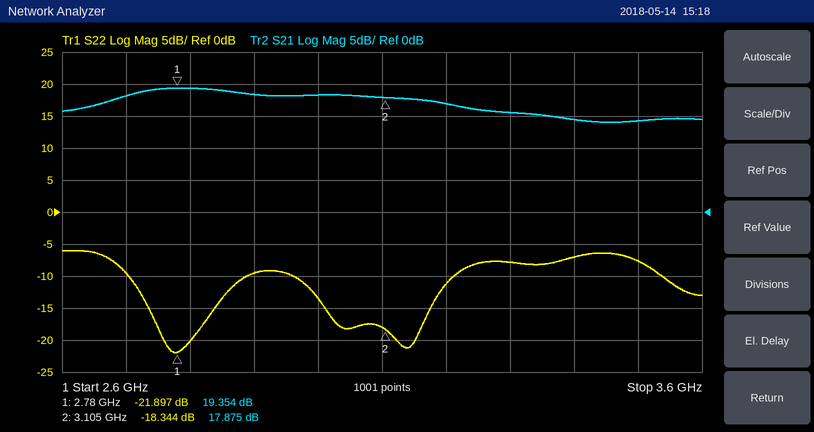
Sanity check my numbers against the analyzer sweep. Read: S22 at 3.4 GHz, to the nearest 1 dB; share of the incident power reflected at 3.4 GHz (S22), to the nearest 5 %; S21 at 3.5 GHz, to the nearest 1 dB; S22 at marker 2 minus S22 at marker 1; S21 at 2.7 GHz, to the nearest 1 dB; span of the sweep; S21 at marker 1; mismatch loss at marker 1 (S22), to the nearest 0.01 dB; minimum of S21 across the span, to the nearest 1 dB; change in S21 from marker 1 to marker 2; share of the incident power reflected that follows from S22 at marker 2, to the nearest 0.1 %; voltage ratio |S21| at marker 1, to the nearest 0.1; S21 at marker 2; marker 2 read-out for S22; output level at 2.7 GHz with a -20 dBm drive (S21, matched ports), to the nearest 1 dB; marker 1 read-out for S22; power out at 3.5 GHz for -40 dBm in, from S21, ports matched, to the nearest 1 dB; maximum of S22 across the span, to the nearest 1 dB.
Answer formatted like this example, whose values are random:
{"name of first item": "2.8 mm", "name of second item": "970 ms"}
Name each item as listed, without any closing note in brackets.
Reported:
{"S22 at 3.4 GHz, to the nearest 1 dB": "-7 dB", "share of the incident power reflected at 3.4 GHz (S22), to the nearest 5 %": "20 %", "S21 at 3.5 GHz, to the nearest 1 dB": "14 dB", "S22 at marker 2 minus S22 at marker 1": "3.553 dB", "S21 at 2.7 GHz, to the nearest 1 dB": "18 dB", "span of the sweep": "1 GHz", "S21 at marker 1": "19.354 dB", "mismatch loss at marker 1 (S22), to the nearest 0.01 dB": "0.03 dB", "minimum of S21 across the span, to the nearest 1 dB": "14 dB", "change in S21 from marker 1 to marker 2": "-1.479 dB", "share of the incident power reflected that follows from S22 at marker 2, to the nearest 0.1 %": "1.5 %", "voltage ratio |S21| at marker 1, to the nearest 0.1": "9.3", "S21 at marker 2": "17.875 dB", "marker 2 read-out for S22": "-18.344 dB", "output level at 2.7 GHz with a -20 dBm drive (S21, matched ports), to the nearest 1 dB": "-2 dBm", "marker 1 read-out for S22": "-21.897 dB", "power out at 3.5 GHz for -40 dBm in, from S21, ports matched, to the nearest 1 dB": "-26 dBm", "maximum of S22 across the span, to the nearest 1 dB": "-6 dB"}
